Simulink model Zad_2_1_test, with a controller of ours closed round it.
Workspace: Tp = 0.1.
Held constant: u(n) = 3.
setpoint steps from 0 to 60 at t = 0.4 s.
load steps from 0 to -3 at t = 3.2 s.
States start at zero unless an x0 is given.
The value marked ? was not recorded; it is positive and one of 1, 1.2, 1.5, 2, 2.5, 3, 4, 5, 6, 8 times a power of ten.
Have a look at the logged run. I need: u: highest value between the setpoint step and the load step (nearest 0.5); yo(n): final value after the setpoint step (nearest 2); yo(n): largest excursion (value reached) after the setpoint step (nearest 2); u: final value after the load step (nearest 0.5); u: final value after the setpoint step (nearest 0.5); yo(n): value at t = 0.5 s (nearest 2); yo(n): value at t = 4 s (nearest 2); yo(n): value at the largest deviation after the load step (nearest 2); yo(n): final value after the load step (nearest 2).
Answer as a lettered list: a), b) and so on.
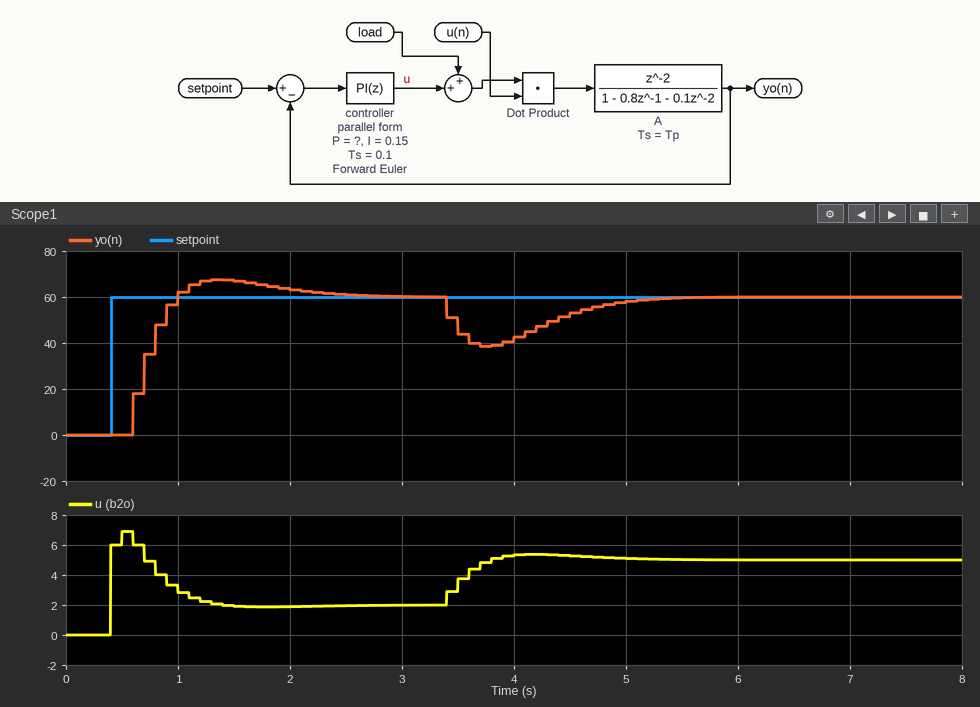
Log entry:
a) 7.0
b) 60
c) 68
d) 5.0
e) 2.0
f) 0
g) 42
h) 38
i) 60
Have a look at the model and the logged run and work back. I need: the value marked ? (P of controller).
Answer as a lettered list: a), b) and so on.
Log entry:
a) 0.1
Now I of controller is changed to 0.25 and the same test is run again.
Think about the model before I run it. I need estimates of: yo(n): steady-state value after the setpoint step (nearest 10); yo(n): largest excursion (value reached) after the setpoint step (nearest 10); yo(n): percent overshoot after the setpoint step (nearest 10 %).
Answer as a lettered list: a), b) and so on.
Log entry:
a) 60
b) 80
c) 30 %
